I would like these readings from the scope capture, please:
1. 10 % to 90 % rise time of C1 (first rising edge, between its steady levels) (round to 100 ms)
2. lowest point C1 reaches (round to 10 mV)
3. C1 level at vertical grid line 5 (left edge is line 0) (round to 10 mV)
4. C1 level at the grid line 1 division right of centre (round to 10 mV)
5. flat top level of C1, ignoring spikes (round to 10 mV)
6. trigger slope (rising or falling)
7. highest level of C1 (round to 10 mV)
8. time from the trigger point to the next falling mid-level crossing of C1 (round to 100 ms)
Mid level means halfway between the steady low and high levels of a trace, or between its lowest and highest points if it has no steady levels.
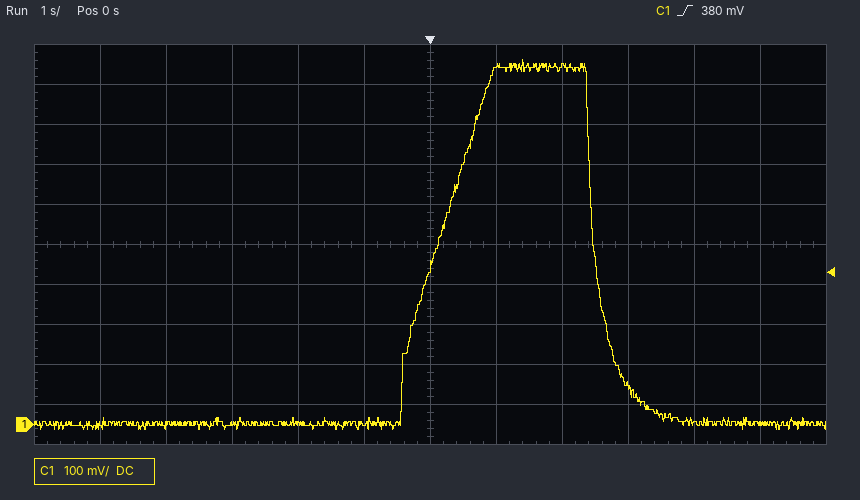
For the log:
1.2 s
-10 mV
0 mV
890 mV
890 mV
rising
910 mV
2.5 s
